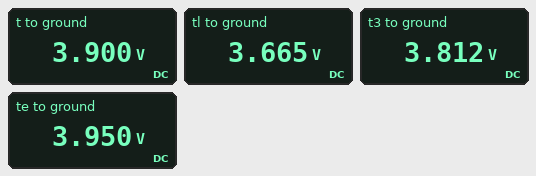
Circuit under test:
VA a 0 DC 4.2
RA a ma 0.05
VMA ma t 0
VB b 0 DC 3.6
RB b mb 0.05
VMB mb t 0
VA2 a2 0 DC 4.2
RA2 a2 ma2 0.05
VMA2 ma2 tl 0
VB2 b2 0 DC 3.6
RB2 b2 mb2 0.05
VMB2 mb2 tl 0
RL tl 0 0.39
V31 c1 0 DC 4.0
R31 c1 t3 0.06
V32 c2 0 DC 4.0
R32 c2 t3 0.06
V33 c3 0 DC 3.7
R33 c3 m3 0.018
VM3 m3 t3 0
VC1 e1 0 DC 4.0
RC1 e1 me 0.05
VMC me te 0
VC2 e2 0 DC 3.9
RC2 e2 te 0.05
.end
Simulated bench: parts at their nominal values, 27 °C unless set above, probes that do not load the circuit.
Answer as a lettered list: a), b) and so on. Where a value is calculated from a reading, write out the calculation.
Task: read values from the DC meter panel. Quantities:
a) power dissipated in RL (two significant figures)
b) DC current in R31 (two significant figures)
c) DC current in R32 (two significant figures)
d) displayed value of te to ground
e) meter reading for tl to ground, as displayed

a) (3.665 V)^2 / 390 mΩ = 34 W
b) (4 V - 3.812 V) / 60 mΩ = 3.1 A
c) (4 V - 3.812 V) / 60 mΩ = 3.1 A
d) 3.950 V
e) 3.665 V
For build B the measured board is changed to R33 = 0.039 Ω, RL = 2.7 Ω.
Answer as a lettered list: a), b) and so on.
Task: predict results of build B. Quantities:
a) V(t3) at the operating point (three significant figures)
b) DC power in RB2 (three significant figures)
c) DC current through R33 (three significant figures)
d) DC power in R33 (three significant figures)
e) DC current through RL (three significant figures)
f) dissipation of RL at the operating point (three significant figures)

a) 3.87 V
b) 1.40 W
c) 4.35 A
d) 737 mW
e) 1.43 A
f) 5.53 W
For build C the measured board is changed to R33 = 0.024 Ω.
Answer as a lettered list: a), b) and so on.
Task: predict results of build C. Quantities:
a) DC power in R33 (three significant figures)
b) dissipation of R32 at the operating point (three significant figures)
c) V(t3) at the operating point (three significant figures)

a) 741 mW
b) 463 mW
c) 3.83 V
